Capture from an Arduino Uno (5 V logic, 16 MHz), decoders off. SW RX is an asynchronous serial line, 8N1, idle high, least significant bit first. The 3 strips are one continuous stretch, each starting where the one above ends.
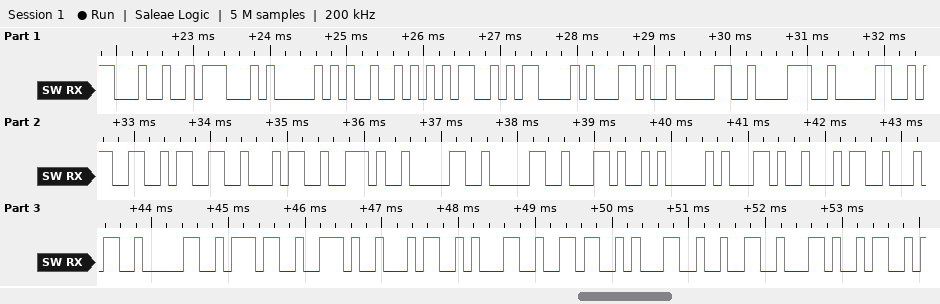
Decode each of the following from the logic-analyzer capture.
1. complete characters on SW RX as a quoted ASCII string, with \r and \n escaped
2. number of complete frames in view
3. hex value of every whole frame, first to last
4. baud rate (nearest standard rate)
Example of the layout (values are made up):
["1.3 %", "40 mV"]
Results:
["\"$GPRMC,080334.00,A,4407.41612,\"", "30", "24 47 50 52 4D 43 2C 30 38 30 33 33 34 2E 30 30 2C 41 2C 34 34 30 37 2E 34 31 36 31 32 2C", "9600 baud"]
